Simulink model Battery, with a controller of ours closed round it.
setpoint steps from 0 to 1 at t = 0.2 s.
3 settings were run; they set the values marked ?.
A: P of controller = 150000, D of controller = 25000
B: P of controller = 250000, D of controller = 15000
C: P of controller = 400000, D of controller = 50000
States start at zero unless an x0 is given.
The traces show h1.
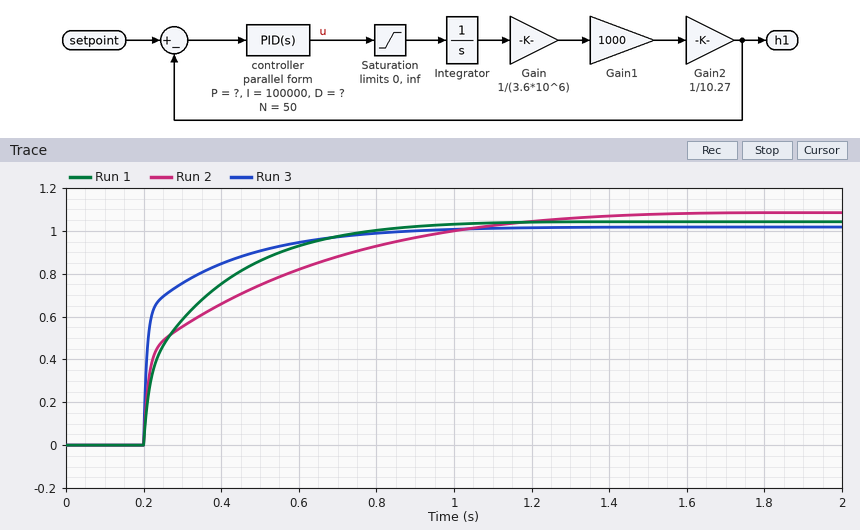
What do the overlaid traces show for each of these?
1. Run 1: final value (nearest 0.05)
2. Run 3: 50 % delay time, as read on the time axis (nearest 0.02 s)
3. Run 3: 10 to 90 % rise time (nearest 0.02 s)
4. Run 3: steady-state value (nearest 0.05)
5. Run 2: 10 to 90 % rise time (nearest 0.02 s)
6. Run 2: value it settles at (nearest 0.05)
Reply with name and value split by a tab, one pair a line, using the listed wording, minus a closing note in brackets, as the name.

Run 1: final value	1.05
Run 3: 50 % delay time, as read on the time axis	0.22 s
Run 3: 10 to 90 % rise time	0.32 s
Run 3: steady-state value	1.00
Run 2: 10 to 90 % rise time	0.72 s
Run 2: value it settles at	1.10
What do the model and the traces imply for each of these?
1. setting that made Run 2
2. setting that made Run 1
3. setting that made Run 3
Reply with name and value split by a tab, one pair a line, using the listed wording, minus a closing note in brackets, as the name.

setting that made Run 2	A
setting that made Run 1	B
setting that made Run 3	C
